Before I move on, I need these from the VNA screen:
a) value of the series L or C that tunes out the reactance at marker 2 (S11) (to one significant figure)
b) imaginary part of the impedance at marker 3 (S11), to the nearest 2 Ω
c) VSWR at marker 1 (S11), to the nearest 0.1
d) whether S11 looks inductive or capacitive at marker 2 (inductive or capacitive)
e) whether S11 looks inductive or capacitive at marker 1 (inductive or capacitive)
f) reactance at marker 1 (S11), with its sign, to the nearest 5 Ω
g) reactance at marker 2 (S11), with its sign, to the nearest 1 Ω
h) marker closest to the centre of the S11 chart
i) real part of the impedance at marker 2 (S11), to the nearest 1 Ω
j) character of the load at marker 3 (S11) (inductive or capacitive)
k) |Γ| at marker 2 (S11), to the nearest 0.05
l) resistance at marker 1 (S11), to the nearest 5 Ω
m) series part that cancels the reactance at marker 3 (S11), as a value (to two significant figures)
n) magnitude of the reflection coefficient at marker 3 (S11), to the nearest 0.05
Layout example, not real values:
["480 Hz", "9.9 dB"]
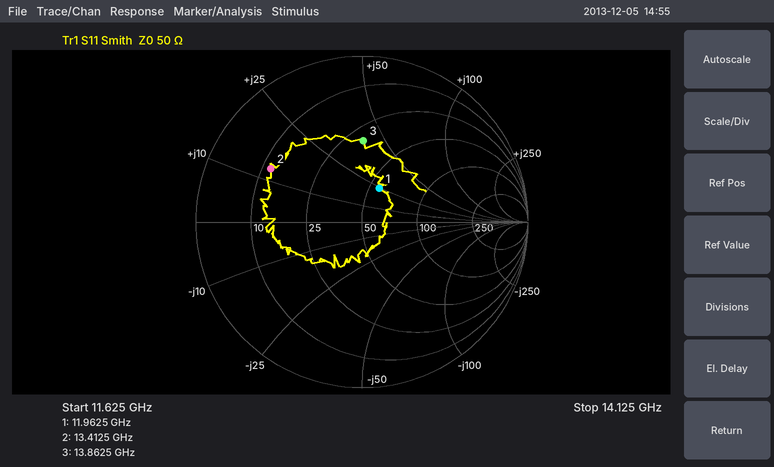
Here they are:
["900 fF", "+40 Ω", "1.6", "inductive", "inductive", "+25 Ω", "+13 Ω", "marker 1", "12 Ω", "inductive", "0.65", "55 Ω", "290 fF", "0.50"]
